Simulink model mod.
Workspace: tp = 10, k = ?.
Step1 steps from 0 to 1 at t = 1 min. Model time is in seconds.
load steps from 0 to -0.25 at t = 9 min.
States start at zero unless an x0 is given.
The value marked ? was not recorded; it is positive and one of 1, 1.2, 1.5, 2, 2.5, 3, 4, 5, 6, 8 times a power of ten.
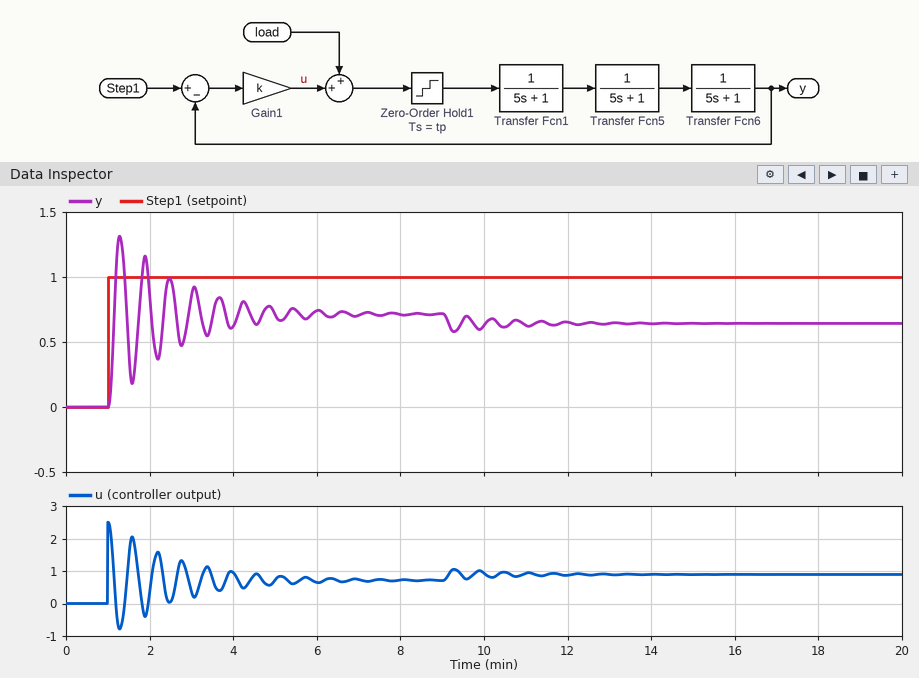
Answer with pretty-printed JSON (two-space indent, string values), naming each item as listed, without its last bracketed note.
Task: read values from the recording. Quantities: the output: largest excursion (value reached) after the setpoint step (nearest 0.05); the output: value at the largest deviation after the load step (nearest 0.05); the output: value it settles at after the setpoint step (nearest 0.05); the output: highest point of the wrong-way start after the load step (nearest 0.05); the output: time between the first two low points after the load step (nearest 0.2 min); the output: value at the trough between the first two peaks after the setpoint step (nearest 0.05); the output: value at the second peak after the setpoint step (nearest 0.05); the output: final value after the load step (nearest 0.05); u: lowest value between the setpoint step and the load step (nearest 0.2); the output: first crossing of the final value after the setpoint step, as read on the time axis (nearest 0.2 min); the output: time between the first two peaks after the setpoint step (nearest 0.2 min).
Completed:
{
  "the output: largest excursion (value reached) after the setpoint step": "1.30",
  "the output: value at the largest deviation after the load step": "0.60",
  "the output: value it settles at after the setpoint step": "0.70",
  "the output: highest point of the wrong-way start after the load step": "0.70",
  "the output: time between the first two low points after the load step": "0.6 min",
  "the output: value at the trough between the first two peaks after the setpoint step": "0.20",
  "the output: value at the second peak after the setpoint step": "1.15",
  "the output: final value after the load step": "0.65",
  "u: lowest value between the setpoint step and the load step": "-0.8",
  "the output: first crossing of the final value after the setpoint step, as read on the time axis": "1.2 min",
  "the output: time between the first two peaks after the setpoint step": "0.6 min"
}
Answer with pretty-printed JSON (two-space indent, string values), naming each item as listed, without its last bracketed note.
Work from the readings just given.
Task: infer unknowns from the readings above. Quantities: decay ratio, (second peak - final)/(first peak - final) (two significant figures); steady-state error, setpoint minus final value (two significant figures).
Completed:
{
  "decay ratio, (second peak - final)/(first peak - final)": "0.75",
  "steady-state error, setpoint minus final value": "0.30"
}
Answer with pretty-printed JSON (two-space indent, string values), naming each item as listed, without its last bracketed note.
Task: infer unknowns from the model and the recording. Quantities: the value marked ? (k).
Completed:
{
  "the value marked ?": "2.5"
}
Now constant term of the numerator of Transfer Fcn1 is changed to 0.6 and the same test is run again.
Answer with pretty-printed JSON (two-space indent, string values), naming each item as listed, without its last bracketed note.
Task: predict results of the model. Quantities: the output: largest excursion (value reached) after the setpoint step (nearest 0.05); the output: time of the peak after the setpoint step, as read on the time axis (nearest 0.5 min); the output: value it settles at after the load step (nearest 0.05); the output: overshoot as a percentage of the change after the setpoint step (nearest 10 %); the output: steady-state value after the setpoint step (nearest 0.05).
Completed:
{
  "the output: largest excursion (value reached) after the setpoint step": "0.90",
  "the output: time of the peak after the setpoint step, as read on the time axis": "1.5 min",
  "the output: value it settles at after the load step": "0.55",
  "the output: overshoot as a percentage of the change after the setpoint step": "50 %",
  "the output: steady-state value after the setpoint step": "0.60"
}
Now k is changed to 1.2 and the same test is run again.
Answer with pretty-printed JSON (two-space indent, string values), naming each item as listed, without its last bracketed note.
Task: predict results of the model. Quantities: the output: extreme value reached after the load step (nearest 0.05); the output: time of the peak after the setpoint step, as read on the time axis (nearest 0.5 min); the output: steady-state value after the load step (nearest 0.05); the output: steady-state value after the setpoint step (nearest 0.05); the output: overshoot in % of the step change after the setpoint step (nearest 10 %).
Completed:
{
  "the output: extreme value reached after the load step": "0.40",
  "the output: time of the peak after the setpoint step, as read on the time axis": "1.5 min",
  "the output: steady-state value after the load step": "0.45",
  "the output: steady-state value after the setpoint step": "0.55",
  "the output: overshoot in % of the step change after the setpoint step": "40 %"
}
